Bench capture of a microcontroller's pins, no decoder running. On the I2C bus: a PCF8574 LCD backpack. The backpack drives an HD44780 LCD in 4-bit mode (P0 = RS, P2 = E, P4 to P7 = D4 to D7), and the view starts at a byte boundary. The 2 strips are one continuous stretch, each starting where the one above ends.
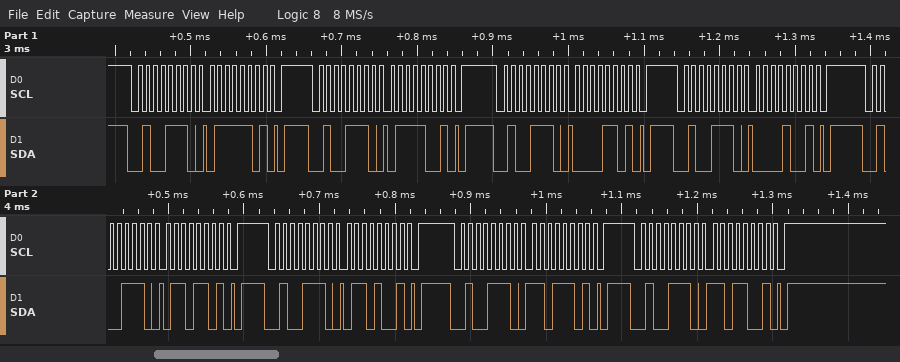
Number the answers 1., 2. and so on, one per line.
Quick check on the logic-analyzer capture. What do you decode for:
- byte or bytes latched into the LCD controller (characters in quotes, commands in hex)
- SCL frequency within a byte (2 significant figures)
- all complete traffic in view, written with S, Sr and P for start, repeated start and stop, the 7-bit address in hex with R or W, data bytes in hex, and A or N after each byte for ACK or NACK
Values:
1. 'p' 'm'
2. 100 kHz
3. S 27W A 7D A P S 27W A 79 A P S 27W A 0D A P S 27W A 09 A P S 27W A 6D A P S 27W A 69 A P S 27W A DD A P S 27W A D9 A P
